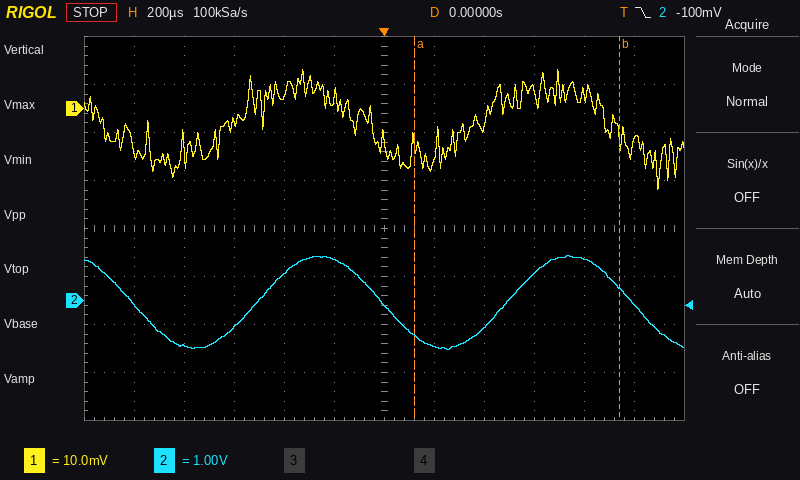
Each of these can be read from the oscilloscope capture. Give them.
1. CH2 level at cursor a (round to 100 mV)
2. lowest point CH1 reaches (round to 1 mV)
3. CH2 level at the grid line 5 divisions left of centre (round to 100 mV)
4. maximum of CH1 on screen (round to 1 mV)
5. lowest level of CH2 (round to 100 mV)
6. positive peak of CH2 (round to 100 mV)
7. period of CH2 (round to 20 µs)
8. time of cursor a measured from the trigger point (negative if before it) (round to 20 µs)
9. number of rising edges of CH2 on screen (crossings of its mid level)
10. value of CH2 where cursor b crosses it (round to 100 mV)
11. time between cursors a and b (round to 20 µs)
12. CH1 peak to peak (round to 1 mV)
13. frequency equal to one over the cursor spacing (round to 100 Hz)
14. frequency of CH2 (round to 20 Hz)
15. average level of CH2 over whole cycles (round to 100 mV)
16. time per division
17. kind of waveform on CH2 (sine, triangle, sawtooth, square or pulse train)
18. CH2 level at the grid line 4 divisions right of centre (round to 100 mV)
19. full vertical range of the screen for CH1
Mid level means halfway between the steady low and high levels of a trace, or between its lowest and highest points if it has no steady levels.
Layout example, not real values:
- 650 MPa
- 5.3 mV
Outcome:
- -700 mV
- -17 mV
- -100 mV
- 8 mV
- -1.0 V
- 900 mV
- 1.00 ms
- +120 µs
- 2
- 300 mV
- 820 µs
- 25 mV
- 1.2 kHz
- 1.00 kHz
- 0.0 V
- 200 µs
- sine
- 900 mV
- 80 mV
